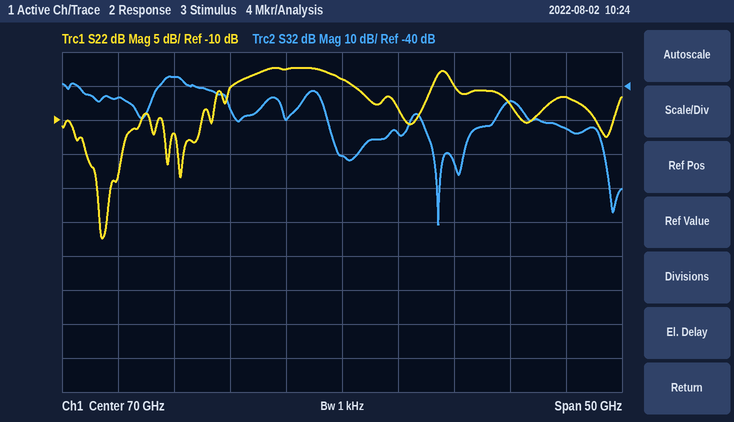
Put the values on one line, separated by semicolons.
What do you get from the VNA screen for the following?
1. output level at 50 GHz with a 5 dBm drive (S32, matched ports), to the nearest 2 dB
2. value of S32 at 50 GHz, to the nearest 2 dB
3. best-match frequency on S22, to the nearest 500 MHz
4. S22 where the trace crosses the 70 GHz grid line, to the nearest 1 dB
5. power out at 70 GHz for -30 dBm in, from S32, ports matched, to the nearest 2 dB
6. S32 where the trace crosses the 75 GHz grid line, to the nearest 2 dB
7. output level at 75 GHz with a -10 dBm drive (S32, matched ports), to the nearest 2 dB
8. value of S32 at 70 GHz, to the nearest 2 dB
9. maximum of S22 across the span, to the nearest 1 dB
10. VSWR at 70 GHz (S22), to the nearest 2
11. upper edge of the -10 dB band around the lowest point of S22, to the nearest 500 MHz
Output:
-38 dBm; -44 dB; 48.5 GHz; -4 dB; -90 dBm; -54 dB; -64 dBm; -60 dB; -2 dB; 4; 52.0 GHz
